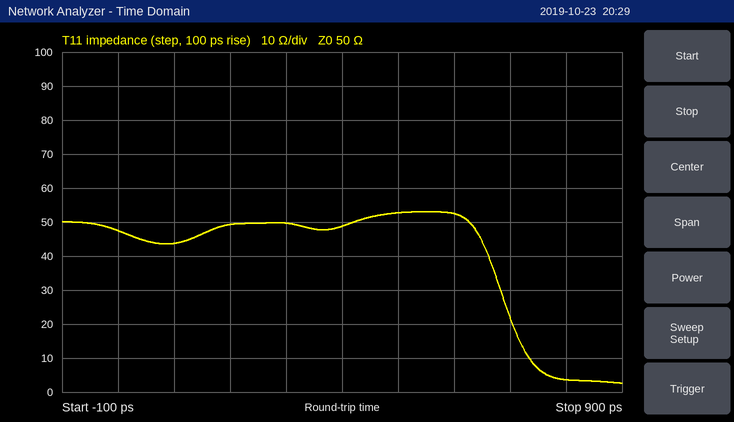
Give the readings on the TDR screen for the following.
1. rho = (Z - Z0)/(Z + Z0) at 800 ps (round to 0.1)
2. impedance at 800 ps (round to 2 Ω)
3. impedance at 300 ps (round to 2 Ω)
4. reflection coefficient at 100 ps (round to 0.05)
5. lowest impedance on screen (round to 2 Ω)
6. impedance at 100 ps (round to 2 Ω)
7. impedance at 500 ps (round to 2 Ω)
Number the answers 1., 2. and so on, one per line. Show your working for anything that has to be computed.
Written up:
1. (4 − 50)/(4 + 50) ≈ -0.9
2. 4 Ω
3. 50 Ω
4. (44 − 50)/(44 + 50) ≈ -0.0638, so -0.05 to the nearest 0.05
5. 2 Ω
6. 44 Ω
7. 52 Ω
